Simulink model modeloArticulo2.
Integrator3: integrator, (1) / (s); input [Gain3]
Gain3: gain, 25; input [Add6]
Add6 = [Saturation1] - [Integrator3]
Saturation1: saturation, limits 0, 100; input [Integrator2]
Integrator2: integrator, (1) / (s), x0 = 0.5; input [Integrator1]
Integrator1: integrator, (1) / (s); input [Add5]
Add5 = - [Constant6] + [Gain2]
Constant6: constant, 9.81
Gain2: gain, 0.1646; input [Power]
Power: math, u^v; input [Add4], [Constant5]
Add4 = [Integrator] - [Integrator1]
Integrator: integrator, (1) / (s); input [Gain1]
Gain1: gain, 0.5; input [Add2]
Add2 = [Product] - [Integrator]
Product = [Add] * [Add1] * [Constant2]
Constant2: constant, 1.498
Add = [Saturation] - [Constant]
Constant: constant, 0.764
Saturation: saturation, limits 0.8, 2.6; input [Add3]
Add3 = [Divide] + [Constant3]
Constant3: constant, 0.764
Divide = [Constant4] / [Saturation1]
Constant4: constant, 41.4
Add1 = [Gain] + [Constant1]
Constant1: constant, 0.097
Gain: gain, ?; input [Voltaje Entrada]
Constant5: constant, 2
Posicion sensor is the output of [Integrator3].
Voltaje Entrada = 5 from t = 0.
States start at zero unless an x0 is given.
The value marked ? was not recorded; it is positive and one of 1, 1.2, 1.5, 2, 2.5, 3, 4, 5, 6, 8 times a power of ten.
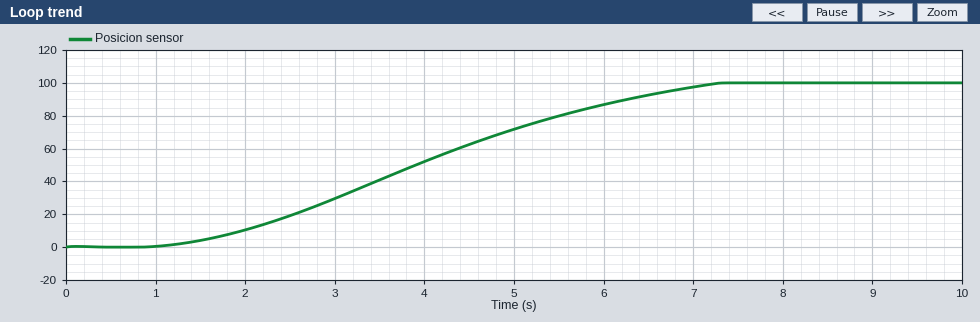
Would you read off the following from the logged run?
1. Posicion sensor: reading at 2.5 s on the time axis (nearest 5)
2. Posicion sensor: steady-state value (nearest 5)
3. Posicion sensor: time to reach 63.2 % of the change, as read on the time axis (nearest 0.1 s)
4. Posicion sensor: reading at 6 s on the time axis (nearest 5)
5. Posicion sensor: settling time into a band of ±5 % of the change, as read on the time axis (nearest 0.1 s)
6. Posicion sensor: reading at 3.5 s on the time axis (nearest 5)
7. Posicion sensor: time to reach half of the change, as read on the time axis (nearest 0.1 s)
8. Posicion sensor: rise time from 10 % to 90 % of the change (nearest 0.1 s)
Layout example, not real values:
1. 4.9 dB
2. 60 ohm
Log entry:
1. 20
2. 100
3. 4.5 s
4. 85
5. 6.7 s
6. 40
7. 3.9 s
8. 4.3 s
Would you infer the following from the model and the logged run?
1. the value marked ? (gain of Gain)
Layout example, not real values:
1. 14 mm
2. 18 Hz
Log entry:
1. 3
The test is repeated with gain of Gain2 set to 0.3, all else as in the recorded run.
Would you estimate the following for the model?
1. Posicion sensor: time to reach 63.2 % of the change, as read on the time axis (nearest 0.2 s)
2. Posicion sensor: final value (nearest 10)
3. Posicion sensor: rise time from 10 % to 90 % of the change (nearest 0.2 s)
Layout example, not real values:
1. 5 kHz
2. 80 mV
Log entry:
1. 4.2 s
2. 100
3. 4.0 s
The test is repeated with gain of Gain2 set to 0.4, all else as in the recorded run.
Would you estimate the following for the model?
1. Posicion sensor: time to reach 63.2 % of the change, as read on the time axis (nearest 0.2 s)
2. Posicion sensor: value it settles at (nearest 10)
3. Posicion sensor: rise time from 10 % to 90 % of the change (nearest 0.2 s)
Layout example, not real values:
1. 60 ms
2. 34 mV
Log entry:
1. 4.0 s
2. 100
3. 4.0 s
